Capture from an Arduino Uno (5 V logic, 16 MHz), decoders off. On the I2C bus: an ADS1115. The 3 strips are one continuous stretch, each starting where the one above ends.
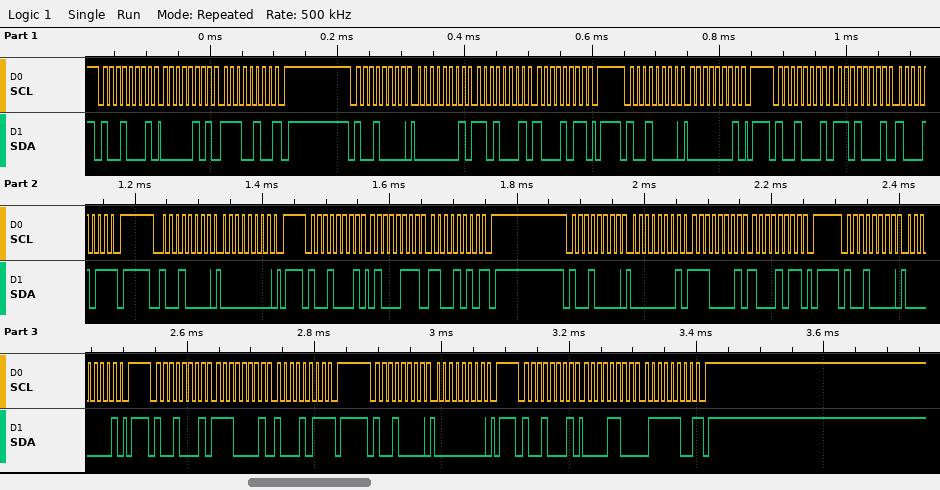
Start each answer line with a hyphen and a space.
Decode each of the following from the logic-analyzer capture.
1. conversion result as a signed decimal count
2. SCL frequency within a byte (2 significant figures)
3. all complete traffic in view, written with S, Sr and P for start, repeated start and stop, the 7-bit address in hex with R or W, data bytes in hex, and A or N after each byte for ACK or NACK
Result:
- 18378
- 100 kHz
- S 48R A 05 A E4 N P S 48W A 01 A D1 A 8B A P S 48W A 01 A P S 48R A D1 A 8B N P S 48W A 00 A P S 48R A 47 A CA N P S 48W A 01 A E1 A 8B A P S 48W A 01 A P S 48R A E1 A 8B N P S 48W A 00 A P S 48R A 0C A 7C N P
